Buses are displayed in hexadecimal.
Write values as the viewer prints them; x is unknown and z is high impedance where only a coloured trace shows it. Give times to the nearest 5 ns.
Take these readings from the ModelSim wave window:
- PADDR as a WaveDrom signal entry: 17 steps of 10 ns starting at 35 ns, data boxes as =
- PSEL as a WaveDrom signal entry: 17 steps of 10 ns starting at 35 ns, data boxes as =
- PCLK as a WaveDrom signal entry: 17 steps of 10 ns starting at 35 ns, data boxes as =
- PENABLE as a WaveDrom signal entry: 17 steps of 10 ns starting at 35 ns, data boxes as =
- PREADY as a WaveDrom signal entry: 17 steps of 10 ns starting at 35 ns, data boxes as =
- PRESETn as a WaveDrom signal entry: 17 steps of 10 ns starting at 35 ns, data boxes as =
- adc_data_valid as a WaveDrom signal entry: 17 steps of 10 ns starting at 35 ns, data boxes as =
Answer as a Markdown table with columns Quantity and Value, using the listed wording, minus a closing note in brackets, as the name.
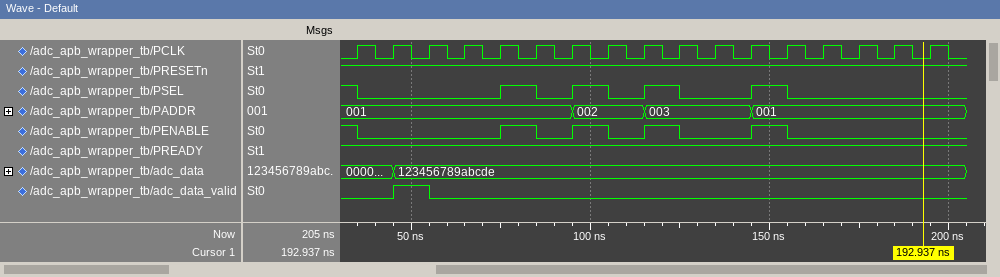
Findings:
| Quantity | Value |
|---|---|
| PADDR as a WaveDrom signal entry: 17 steps of 10 ns starting at 35 ns, data boxes as = | {name: 'PADDR', wave: '=.....=.=..=.....', data: '001 002 003 001'} |
| PSEL as a WaveDrom signal entry: 17 steps of 10 ns starting at 35 ns, data boxes as = | {name: 'PSEL', wave: '0...101010.10....'} |
| PCLK as a WaveDrom signal entry: 17 steps of 10 ns starting at 35 ns, data boxes as = | {name: 'PCLK', wave: 'p................'} |
| PENABLE as a WaveDrom signal entry: 17 steps of 10 ns starting at 35 ns, data boxes as = | {name: 'PENABLE', wave: '0...101010.10....'} |
| PREADY as a WaveDrom signal entry: 17 steps of 10 ns starting at 35 ns, data boxes as = | {name: 'PREADY', wave: '1................'} |
| PRESETn as a WaveDrom signal entry: 17 steps of 10 ns starting at 35 ns, data boxes as = | {name: 'PRESETn', wave: '1................'} |
| adc_data_valid as a WaveDrom signal entry: 17 steps of 10 ns starting at 35 ns, data boxes as = | {name: 'adc_data_valid', wave: '010..............'} |
